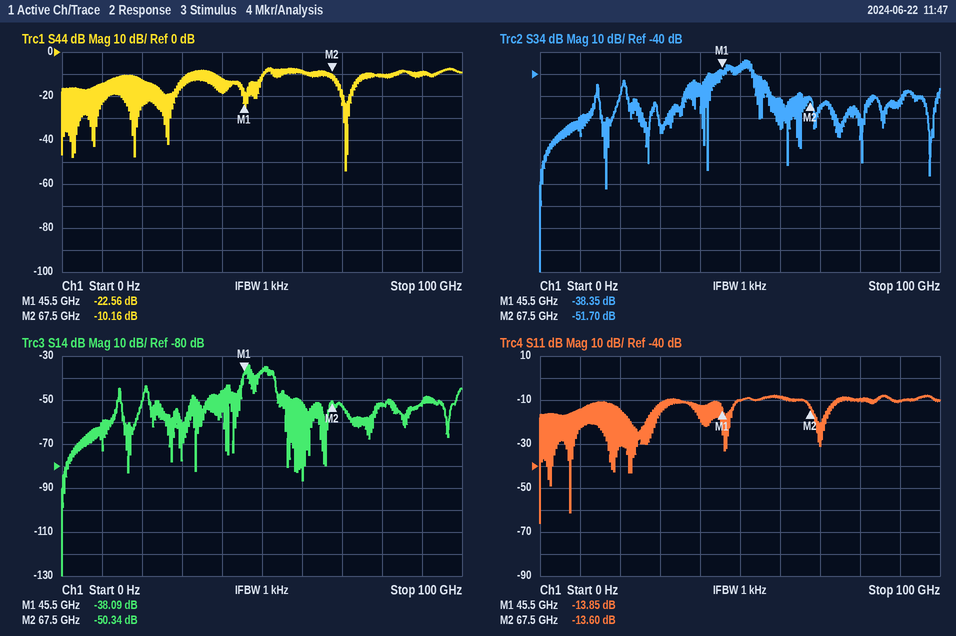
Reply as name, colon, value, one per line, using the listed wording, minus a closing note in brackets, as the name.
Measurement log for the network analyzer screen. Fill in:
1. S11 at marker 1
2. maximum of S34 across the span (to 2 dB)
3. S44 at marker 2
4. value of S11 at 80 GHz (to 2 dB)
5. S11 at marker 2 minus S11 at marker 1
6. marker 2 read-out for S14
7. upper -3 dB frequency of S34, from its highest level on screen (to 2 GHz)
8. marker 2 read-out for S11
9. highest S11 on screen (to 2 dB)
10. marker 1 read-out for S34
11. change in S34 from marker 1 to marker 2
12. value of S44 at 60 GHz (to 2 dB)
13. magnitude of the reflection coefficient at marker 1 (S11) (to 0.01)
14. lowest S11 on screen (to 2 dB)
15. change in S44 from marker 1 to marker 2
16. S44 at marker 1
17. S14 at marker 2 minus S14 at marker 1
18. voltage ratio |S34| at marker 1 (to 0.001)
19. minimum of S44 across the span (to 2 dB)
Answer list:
S11 at marker 1: -13.85 dB
maximum of S34 across the span: -34 dB
S44 at marker 2: -10.16 dB
value of S11 at 80 GHz: -10 dB
S11 at marker 2 minus S11 at marker 1: 0.25 dB
marker 2 read-out for S14: -50.34 dB
upper -3 dB frequency of S34, from its highest level on screen: 52 GHz
marker 2 read-out for S11: -13.60 dB
highest S11 on screen: -8 dB
marker 1 read-out for S34: -38.35 dB
change in S34 from marker 1 to marker 2: -13.35 dB
value of S44 at 60 GHz: -8 dB
magnitude of the reflection coefficient at marker 1 (S11): 0.20
lowest S11 on screen: -66 dB
change in S44 from marker 1 to marker 2: 12.40 dB
S44 at marker 1: -22.56 dB
S14 at marker 2 minus S14 at marker 1: -12.25 dB
voltage ratio |S34| at marker 1: 0.012
minimum of S44 across the span: -54 dB
